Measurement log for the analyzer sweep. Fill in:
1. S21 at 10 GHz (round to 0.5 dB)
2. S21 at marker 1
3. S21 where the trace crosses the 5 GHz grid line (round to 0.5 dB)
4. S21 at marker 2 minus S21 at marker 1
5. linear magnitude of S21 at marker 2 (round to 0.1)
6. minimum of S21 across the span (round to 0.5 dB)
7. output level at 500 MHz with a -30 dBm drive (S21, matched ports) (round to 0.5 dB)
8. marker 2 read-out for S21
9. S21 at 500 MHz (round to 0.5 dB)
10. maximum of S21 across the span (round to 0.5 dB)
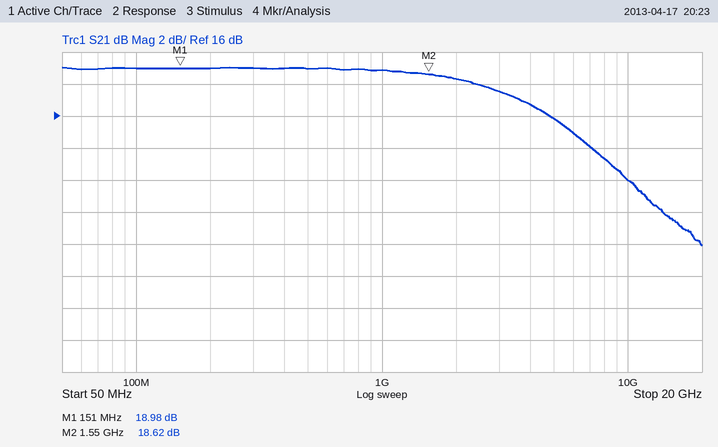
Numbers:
12.0 dB
18.98 dB
16.0 dB
-0.36 dB
8.5
8.0 dB
-11.0 dBm
18.62 dB
19.0 dB
19.0 dB
